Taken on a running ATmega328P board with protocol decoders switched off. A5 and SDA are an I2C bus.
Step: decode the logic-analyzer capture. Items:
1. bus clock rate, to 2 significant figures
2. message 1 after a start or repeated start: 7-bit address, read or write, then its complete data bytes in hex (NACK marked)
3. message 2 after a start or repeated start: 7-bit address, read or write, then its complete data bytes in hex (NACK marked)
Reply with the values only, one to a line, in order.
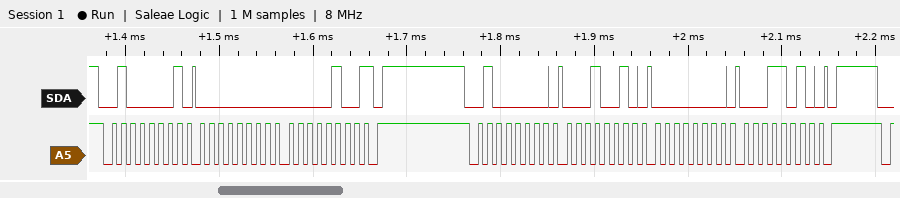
100 kHz
0x20 read: 00 04 NACK
0x20 write: 12 00 1A
